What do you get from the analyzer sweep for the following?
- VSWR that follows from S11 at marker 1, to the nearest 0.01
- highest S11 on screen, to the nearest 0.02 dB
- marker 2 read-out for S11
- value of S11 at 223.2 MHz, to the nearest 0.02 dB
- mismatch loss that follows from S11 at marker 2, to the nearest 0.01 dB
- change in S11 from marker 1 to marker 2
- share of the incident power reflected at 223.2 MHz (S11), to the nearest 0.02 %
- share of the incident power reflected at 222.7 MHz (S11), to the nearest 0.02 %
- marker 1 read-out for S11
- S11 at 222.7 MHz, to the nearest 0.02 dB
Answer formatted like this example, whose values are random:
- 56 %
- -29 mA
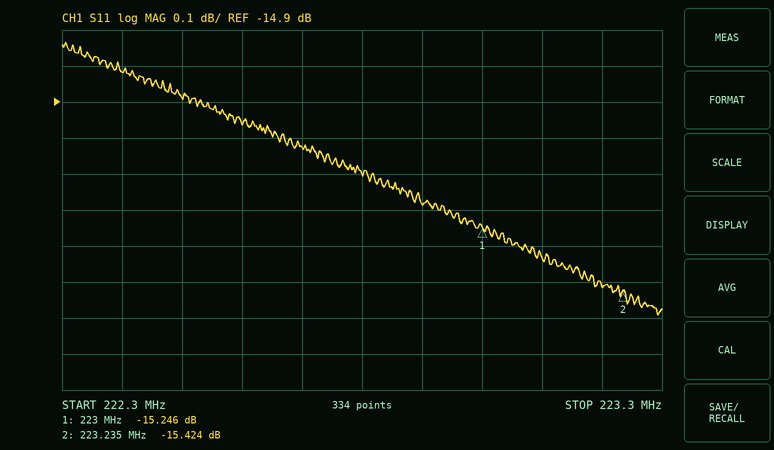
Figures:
- 1.42
- -14.74 dB
- -15.424 dB
- -15.42 dB
- 0.13 dB
- -0.178 dB
- 2.88 %
- 3.14 %
- -15.246 dB
- -15.02 dB
